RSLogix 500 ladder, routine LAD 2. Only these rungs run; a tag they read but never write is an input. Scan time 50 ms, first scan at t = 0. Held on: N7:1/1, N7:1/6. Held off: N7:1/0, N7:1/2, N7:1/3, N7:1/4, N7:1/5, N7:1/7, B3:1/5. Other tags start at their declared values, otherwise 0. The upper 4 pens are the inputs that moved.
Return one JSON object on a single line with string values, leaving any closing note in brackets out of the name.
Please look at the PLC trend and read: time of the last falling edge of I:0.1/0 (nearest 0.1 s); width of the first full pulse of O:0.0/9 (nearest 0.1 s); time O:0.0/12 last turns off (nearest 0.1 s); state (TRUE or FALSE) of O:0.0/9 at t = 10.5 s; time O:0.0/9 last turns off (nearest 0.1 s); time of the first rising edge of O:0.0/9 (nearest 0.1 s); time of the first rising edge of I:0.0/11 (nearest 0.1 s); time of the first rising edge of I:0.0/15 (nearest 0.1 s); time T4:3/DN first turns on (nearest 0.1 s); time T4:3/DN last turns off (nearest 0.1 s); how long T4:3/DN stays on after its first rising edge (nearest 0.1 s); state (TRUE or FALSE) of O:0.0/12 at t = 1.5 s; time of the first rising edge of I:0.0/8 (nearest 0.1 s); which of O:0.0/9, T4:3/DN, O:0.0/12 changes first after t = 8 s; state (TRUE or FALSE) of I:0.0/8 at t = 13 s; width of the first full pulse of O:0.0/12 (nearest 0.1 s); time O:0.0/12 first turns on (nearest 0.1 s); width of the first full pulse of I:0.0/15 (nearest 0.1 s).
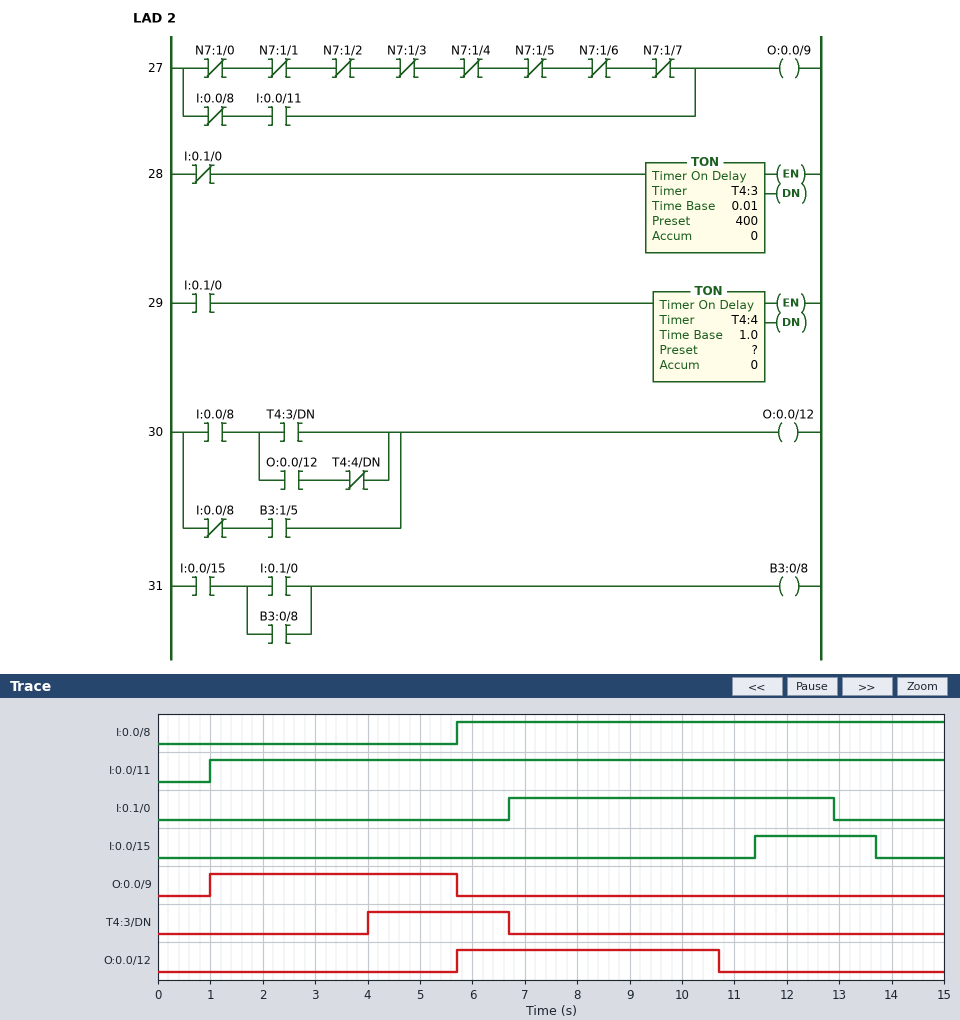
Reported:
{"time of the last falling edge of I:0.1/0": "12.9 s", "width of the first full pulse of O:0.0/9": "4.7 s", "time O:0.0/12 last turns off": "10.7 s", "state (TRUE or FALSE) of O:0.0/9 at t = 10.5 s": "FALSE", "time O:0.0/9 last turns off": "5.7 s", "time of the first rising edge of O:0.0/9": "1.0 s", "time of the first rising edge of I:0.0/11": "1.0 s", "time of the first rising edge of I:0.0/15": "11.4 s", "time T4:3/DN first turns on": "4.0 s", "time T4:3/DN last turns off": "6.7 s", "how long T4:3/DN stays on after its first rising edge": "2.7 s", "state (TRUE or FALSE) of O:0.0/12 at t = 1.5 s": "FALSE", "time of the first rising edge of I:0.0/8": "5.7 s", "which of O:0.0/9, T4:3/DN, O:0.0/12 changes first after t = 8 s": "O:0.0/12", "state (TRUE or FALSE) of I:0.0/8 at t = 13 s": "TRUE", "width of the first full pulse of O:0.0/12": "5.0 s", "time O:0.0/12 first turns on": "5.7 s", "width of the first full pulse of I:0.0/15": "2.3 s"}
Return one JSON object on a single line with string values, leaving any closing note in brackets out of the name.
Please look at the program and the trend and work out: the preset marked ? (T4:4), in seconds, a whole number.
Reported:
{"the preset marked ? (T4:4), in seconds, a whole number": "4 s"}
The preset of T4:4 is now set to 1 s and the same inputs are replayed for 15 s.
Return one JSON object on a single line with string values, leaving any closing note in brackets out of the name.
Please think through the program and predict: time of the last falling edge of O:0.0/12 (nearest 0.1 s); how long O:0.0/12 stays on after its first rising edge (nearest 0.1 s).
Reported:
{"time of the last falling edge of O:0.0/12": "7.7 s", "how long O:0.0/12 stays on after its first rising edge": "2.0 s"}
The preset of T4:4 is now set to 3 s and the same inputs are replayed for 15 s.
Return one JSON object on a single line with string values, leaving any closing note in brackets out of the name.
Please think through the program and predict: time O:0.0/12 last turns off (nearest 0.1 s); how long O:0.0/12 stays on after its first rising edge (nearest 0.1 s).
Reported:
{"time O:0.0/12 last turns off": "9.7 s", "how long O:0.0/12 stays on after its first rising edge": "4.0 s"}
